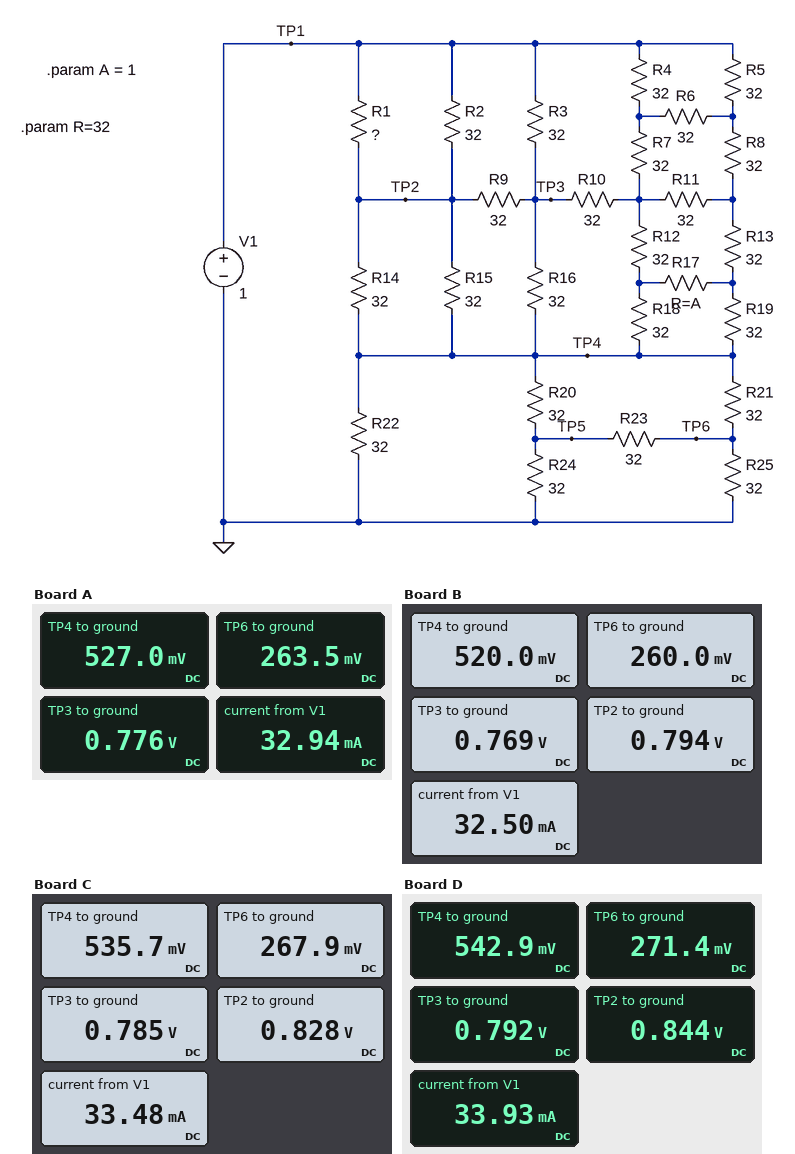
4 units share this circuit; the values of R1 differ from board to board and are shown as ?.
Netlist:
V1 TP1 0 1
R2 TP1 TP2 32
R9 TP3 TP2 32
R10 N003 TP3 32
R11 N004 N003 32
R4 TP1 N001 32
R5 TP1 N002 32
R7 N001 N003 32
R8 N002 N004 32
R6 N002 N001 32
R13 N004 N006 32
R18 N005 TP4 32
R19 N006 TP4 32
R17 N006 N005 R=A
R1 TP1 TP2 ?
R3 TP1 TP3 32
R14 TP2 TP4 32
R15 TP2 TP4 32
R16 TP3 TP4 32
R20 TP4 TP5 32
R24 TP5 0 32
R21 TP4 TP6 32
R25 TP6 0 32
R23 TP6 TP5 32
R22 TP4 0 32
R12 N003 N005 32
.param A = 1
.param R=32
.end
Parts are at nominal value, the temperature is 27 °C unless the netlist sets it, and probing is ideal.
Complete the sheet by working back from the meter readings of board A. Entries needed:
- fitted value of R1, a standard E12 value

15 Ω
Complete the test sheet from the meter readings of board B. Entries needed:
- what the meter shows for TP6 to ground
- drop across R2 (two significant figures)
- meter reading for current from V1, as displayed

260.0 mV
210 mV
32.50 mA
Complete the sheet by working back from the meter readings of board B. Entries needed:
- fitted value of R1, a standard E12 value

18 Ω
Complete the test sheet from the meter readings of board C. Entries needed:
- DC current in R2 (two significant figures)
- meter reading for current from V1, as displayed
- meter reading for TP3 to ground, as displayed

5.4 mA
33.48 mA
0.785 V
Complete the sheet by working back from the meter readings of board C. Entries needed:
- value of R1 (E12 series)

12 Ω
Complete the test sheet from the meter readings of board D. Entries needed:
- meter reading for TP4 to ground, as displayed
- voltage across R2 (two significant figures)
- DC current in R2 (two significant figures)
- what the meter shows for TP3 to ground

542.9 mV
160 mV
4.9 mA
0.792 V
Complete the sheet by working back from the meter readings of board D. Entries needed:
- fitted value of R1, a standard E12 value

10 Ω
